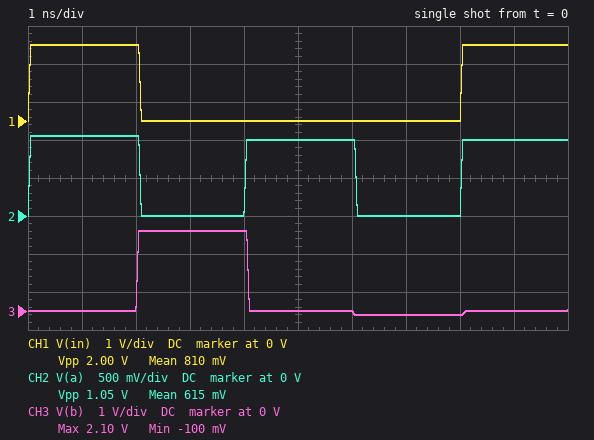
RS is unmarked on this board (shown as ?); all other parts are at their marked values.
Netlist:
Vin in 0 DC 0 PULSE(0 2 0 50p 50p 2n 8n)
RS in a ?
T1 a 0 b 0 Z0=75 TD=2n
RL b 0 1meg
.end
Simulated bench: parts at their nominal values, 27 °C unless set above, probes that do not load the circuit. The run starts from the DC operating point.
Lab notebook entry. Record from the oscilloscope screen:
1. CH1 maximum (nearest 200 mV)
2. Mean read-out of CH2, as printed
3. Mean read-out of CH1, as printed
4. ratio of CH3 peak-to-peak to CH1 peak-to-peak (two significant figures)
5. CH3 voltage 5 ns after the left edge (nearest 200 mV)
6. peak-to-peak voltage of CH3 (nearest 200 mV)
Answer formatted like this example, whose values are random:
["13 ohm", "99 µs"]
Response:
["2.0 V", "615 mV", "810 mV", "1.1", "0 V", "2.2 V"]
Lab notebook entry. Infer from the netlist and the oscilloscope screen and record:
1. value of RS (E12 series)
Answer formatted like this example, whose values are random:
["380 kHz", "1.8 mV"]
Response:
["68 Ω"]
